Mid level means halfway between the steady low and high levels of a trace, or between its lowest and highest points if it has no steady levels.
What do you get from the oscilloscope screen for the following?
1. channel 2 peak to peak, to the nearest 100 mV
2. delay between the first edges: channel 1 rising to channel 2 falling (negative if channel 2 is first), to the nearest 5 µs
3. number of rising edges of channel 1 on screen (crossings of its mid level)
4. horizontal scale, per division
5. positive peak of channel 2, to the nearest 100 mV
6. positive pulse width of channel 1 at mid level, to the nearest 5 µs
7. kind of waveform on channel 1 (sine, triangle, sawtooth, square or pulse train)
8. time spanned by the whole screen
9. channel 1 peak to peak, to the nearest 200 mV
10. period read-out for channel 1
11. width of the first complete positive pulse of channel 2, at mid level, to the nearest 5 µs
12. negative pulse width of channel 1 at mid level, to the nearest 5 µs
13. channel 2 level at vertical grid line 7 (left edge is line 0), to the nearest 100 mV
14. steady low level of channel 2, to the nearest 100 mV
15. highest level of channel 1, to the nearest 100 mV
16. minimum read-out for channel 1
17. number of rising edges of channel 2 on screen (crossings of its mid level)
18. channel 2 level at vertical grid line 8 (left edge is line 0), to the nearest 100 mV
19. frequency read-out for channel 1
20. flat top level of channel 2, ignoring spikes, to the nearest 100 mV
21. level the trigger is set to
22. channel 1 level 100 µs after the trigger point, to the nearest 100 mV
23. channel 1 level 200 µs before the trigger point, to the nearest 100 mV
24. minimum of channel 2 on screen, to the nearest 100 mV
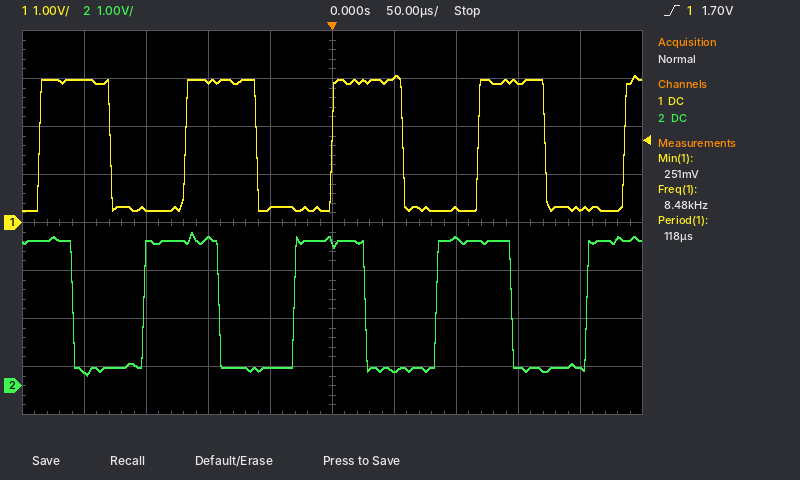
3.0 V
+25 µs
5
50 µs
3.2 V
55 µs
square
500 µs
2.8 V
118 µs
60 µs
60 µs
3.1 V
400 mV
3.1 V
251 mV
4
400 mV
8.48 kHz
3.0 V
1.70 V
300 mV
3.0 V
200 mV
